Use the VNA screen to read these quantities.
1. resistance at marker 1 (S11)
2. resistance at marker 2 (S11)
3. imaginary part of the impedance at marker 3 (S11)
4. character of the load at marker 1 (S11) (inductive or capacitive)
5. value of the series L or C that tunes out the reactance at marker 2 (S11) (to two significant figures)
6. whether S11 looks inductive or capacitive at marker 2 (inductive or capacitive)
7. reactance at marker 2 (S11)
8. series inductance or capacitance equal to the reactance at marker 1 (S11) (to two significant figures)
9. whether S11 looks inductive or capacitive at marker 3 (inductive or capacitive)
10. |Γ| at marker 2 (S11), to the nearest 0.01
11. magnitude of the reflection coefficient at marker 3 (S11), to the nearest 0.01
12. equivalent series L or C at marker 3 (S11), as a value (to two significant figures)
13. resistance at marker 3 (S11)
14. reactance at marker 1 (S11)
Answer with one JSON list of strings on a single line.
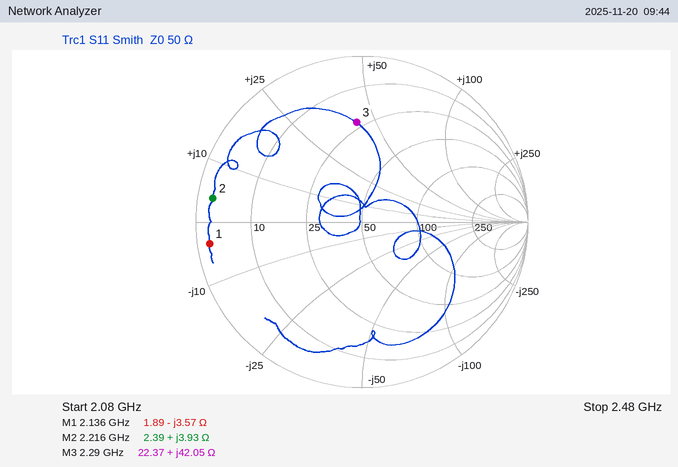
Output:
["1.89 Ω", "2.39 Ω", "+42.05 Ω", "capacitive", "18 pF", "inductive", "+3.93 Ω", "21 pF", "inductive", "0.91", "0.60", "2.9 nH", "22.37 Ω", "-3.57 Ω"]
